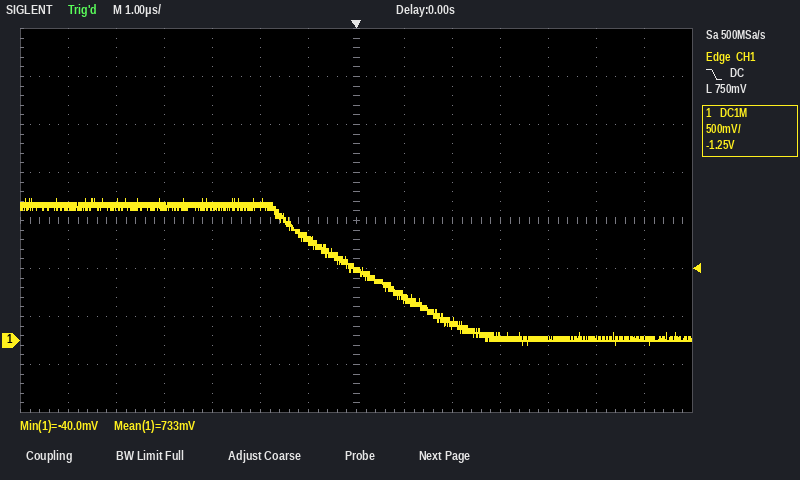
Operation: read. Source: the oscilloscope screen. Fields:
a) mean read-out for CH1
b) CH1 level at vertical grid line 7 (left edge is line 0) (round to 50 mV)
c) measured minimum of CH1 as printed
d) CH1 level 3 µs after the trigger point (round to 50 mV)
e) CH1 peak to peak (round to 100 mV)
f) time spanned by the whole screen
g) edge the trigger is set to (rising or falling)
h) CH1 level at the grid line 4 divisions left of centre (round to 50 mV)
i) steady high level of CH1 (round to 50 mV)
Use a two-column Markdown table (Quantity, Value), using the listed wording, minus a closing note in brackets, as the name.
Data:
| Quantity | Value |
|---|---|
| mean read-out for CH1 | 733 mV |
| CH1 level at vertical grid line 7 (left edge is line 0) | 750 mV |
| measured minimum of CH1 as printed | -40.0 mV |
| CH1 level 3 µs after the trigger point | 50 mV |
| CH1 peak to peak | 1.50 V |
| time spanned by the whole screen | 14 µs |
| edge the trigger is set to | falling |
| CH1 level at the grid line 4 divisions left of centre | 1.40 V |
| steady high level of CH1 | 1.40 V |
